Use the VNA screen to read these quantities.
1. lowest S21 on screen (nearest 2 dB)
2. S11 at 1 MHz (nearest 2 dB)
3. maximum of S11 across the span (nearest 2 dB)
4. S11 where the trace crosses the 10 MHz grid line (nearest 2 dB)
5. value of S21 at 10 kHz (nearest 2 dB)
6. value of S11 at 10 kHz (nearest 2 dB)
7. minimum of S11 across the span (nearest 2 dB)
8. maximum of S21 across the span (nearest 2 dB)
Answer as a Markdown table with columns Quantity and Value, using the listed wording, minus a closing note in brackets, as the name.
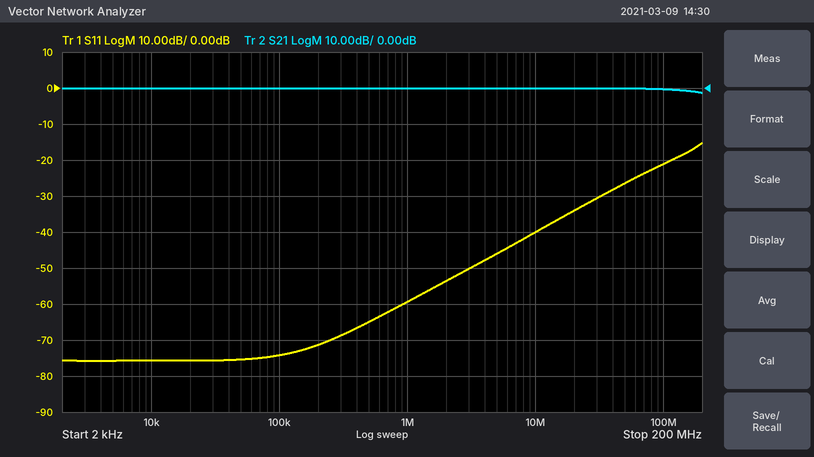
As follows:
| Quantity | Value |
|---|---|
| lowest S21 on screen | -2 dB |
| S11 at 1 MHz | -60 dB |
| maximum of S11 across the span | -16 dB |
| S11 where the trace crosses the 10 MHz grid line | -40 dB |
| value of S21 at 10 kHz | 0 dB |
| value of S11 at 10 kHz | -76 dB |
| minimum of S11 across the span | -76 dB |
| maximum of S21 across the span | 0 dB |
